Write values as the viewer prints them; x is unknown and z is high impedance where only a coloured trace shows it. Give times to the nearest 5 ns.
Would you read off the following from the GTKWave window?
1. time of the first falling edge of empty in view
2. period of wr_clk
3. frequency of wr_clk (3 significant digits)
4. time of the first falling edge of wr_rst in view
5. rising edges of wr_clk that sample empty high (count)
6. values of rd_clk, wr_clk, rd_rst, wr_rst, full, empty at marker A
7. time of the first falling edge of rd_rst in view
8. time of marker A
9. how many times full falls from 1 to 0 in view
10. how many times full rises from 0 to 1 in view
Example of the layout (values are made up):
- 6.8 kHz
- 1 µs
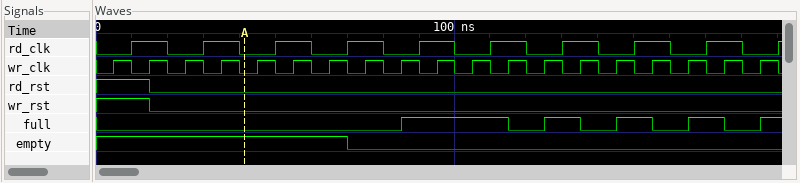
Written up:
- 70 ns
- 10 ns
- 100 MHz
- 15 ns
- 7
- rd_clk=0, wr_clk=0, rd_rst=0, wr_rst=0, full=0, empty=1
- 15 ns
- 40 ns
- 4
- 5
